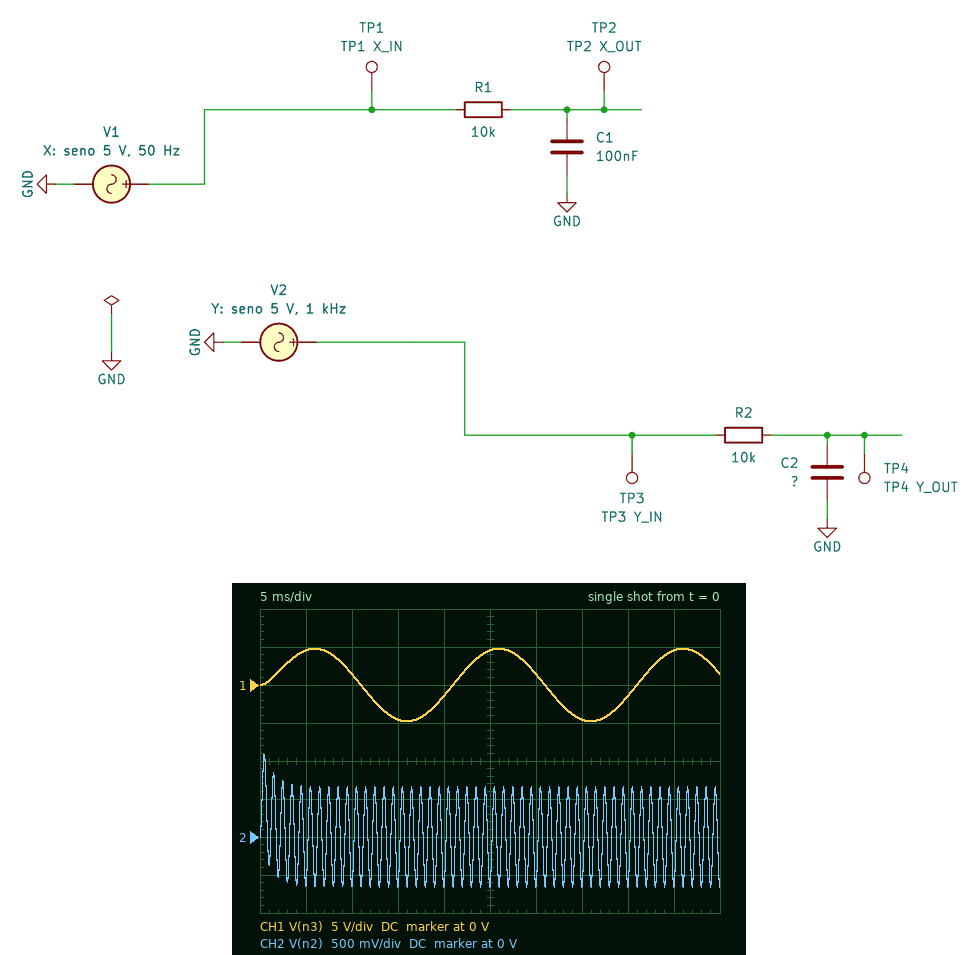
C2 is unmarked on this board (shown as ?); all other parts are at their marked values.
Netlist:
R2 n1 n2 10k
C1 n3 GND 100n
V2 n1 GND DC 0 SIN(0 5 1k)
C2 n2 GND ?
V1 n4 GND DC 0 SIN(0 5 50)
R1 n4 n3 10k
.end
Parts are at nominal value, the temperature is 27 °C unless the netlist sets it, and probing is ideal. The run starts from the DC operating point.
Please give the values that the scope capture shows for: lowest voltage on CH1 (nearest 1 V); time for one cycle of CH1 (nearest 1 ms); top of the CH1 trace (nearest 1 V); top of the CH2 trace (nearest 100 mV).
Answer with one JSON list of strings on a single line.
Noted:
["-5 V", "20 ms", "5 V", "1.1 V"]
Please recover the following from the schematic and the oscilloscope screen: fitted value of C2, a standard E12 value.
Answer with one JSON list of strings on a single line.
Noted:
["120 nF"]
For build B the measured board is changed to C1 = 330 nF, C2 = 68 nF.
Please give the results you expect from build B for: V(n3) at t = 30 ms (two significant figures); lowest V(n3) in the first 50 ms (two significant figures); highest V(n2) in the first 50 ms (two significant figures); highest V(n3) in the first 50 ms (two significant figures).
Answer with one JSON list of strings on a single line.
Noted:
["2.5 V", "-3.5 V", "1.7 V", "3.7 V"]
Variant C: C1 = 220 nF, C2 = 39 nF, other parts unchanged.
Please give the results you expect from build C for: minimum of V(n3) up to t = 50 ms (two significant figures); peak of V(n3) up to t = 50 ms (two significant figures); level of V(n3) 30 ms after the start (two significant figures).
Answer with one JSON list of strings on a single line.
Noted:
["-4.1 V", "4.2 V", "2.3 V"]
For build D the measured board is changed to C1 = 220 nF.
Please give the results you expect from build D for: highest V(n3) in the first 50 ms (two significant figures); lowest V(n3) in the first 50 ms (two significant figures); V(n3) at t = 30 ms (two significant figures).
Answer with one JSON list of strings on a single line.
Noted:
["4.2 V", "-4.1 V", "2.3 V"]
